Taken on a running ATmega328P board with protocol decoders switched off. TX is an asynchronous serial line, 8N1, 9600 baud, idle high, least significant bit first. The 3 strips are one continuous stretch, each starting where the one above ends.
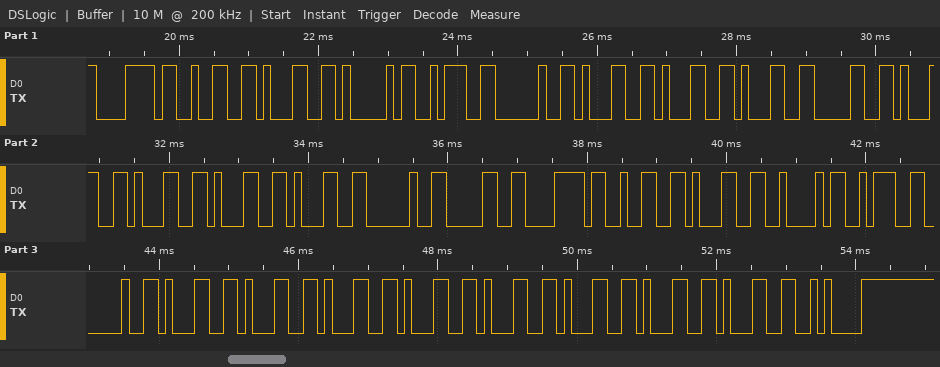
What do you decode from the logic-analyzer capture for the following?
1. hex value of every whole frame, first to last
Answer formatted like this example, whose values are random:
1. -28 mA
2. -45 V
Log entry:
1. 78 32 31 41 3A 20 31 31 31 30 31 31 31 31 20 30 78 32 31 42 3A 20 31 31 31 31 31 31 31 31 0A
